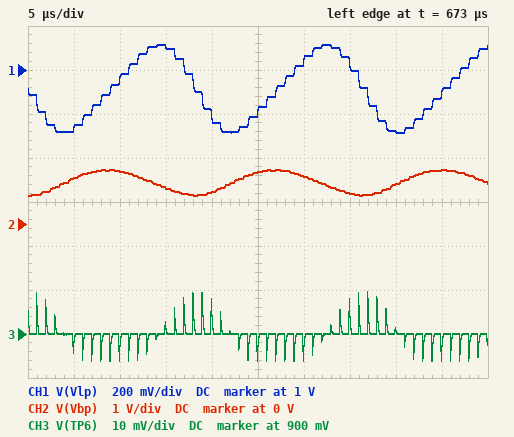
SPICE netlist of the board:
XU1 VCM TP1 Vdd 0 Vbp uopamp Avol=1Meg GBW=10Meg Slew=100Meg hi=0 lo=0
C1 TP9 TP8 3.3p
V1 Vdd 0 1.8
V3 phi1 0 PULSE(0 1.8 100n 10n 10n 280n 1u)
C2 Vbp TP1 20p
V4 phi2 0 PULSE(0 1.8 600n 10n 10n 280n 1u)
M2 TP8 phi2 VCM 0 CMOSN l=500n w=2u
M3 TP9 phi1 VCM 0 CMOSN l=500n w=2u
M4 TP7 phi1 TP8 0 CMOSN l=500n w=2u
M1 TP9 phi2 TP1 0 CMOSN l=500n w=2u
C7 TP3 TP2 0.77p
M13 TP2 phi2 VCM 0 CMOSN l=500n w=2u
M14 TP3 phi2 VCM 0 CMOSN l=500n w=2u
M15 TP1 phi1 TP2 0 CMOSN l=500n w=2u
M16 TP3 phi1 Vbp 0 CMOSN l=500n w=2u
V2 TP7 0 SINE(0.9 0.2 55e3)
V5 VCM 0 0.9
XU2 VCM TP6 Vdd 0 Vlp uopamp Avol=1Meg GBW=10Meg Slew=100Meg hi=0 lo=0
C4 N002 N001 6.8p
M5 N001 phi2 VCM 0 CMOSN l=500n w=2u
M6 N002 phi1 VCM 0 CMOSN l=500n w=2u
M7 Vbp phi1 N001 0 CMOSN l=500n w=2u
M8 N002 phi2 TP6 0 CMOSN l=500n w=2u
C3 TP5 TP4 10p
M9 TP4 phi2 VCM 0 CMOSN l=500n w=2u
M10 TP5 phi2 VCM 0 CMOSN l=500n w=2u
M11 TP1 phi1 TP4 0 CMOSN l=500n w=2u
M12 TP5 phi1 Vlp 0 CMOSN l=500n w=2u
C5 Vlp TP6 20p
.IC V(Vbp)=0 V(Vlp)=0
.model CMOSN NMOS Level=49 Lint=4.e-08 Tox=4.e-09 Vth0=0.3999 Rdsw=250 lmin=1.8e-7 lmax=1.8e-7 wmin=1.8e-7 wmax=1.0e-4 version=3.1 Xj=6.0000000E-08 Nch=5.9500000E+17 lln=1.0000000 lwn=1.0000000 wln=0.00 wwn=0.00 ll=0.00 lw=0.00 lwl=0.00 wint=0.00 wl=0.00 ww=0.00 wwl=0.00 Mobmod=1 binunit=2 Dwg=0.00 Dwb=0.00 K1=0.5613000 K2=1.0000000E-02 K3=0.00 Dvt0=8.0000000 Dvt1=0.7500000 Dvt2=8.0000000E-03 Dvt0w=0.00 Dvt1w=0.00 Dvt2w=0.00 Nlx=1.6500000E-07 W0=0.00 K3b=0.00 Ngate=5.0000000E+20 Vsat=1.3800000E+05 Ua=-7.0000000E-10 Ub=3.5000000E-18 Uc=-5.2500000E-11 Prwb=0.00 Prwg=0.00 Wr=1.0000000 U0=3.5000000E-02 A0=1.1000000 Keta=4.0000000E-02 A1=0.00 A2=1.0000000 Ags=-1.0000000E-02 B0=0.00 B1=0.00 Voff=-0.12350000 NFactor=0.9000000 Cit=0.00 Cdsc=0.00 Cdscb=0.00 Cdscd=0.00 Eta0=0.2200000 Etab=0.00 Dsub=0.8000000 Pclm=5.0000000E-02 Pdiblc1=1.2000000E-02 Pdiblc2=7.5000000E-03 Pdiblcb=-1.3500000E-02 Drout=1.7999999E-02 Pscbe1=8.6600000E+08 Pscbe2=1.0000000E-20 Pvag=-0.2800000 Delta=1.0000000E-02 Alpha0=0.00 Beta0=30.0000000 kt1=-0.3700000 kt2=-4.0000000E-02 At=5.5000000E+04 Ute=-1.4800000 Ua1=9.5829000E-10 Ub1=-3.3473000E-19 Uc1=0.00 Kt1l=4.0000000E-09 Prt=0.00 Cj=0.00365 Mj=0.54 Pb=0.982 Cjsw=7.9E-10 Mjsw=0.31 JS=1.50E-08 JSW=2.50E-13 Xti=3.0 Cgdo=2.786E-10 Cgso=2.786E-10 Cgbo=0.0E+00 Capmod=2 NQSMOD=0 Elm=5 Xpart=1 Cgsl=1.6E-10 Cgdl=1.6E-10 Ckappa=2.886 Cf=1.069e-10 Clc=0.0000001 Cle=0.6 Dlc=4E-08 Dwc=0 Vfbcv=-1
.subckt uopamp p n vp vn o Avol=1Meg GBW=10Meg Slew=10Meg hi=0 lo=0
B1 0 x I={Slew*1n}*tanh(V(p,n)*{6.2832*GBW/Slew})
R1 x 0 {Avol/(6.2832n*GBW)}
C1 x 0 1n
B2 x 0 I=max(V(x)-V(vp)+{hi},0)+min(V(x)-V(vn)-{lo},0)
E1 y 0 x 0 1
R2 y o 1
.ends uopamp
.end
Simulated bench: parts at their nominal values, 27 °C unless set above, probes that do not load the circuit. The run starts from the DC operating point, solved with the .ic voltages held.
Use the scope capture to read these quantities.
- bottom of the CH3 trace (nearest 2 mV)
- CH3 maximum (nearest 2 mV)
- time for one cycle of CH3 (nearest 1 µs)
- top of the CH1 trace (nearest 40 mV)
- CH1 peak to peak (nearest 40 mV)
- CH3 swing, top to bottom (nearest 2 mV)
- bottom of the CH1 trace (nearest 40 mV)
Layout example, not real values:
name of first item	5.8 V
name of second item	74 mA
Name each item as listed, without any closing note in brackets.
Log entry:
bottom of the CH3 trace	894 mV
CH3 maximum	910 mV
time for one cycle of CH3	18 µs
top of the CH1 trace	1.12 V
CH1 peak to peak	400 mV
CH3 swing, top to bottom	16 mV
bottom of the CH1 trace	720 mV
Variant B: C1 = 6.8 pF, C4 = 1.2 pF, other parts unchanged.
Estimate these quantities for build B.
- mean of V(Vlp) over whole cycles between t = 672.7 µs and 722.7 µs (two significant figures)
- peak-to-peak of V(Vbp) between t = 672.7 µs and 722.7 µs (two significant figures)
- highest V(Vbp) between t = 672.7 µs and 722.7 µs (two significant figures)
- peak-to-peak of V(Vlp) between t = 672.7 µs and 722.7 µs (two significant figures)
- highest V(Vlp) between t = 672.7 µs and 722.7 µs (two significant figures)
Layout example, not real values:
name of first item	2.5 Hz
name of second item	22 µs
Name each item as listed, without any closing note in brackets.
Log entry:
mean of V(Vlp) over whole cycles between t = 672.7 µs and 722.7 µs	890 mV
peak-to-peak of V(Vbp) between t = 672.7 µs and 722.7 µs	430 mV
highest V(Vbp) between t = 672.7 µs and 722.7 µs	1.1 V
peak-to-peak of V(Vlp) between t = 672.7 µs and 722.7 µs	71 mV
highest V(Vlp) between t = 672.7 µs and 722.7 µs	930 mV
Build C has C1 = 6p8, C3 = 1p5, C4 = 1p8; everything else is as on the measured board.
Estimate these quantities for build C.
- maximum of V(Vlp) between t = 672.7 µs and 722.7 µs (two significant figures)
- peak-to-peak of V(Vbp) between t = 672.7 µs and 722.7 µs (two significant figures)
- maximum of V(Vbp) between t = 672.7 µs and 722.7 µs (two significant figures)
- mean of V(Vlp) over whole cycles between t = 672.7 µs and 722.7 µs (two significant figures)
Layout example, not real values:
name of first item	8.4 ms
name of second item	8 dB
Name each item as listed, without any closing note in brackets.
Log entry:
maximum of V(Vlp) between t = 672.7 µs and 722.7 µs	890 mV
peak-to-peak of V(Vbp) between t = 672.7 µs and 722.7 µs	360 mV
maximum of V(Vbp) between t = 672.7 µs and 722.7 µs	1.1 V
mean of V(Vlp) over whole cycles between t = 672.7 µs and 722.7 µs	840 mV
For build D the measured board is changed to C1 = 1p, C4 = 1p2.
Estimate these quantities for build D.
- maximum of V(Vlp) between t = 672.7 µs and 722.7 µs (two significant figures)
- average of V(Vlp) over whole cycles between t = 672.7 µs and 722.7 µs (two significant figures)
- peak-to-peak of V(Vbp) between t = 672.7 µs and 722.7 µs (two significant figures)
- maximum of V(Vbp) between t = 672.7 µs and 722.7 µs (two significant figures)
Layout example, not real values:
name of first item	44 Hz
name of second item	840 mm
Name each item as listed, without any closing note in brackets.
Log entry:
maximum of V(Vlp) between t = 672.7 µs and 722.7 µs	910 mV
average of V(Vlp) over whole cycles between t = 672.7 µs and 722.7 µs	900 mV
peak-to-peak of V(Vbp) between t = 672.7 µs and 722.7 µs	73 mV
maximum of V(Vbp) between t = 672.7 µs and 722.7 µs	940 mV
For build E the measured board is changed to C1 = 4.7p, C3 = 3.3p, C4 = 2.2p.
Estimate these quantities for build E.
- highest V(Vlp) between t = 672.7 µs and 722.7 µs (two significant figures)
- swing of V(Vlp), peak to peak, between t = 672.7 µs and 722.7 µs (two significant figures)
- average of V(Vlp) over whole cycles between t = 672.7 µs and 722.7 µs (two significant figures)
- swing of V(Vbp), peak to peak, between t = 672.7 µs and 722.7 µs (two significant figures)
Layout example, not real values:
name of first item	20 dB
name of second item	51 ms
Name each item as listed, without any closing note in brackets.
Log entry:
highest V(Vlp) between t = 672.7 µs and 722.7 µs	930 mV
swing of V(Vlp), peak to peak, between t = 672.7 µs and 722.7 µs	91 mV
average of V(Vlp) over whole cycles between t = 672.7 µs and 722.7 µs	890 mV
swing of V(Vbp), peak to peak, between t = 672.7 µs and 722.7 µs	300 mV
